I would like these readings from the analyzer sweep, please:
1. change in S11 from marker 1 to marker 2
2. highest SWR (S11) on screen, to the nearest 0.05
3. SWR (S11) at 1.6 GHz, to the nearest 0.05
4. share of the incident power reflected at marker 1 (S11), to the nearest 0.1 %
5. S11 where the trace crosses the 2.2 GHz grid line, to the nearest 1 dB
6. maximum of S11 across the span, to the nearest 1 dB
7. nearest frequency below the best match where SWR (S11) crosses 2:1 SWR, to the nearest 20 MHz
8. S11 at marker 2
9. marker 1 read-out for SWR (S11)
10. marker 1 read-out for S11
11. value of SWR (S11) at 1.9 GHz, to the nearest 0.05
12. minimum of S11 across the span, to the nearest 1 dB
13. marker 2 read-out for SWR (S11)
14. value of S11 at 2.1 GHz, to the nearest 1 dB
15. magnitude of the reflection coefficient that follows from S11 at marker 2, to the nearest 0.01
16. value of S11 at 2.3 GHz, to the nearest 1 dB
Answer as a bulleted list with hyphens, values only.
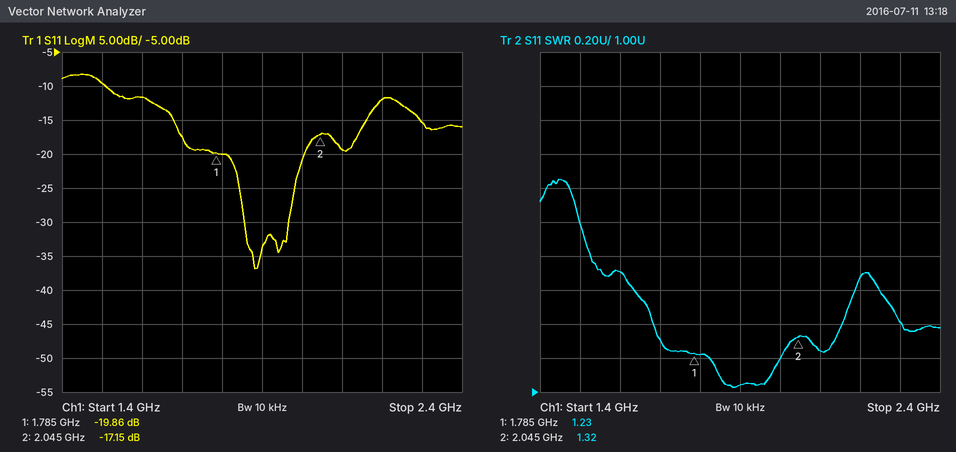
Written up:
- 2.71 dB
- 2.25
- 1.70
- 1.0 %
- -12 dB
- -8 dB
- 1.50 GHz
- -17.15 dB
- 1.23
- -19.86 dB
- 1.05
- -37 dB
- 1.32
- -19 dB
- 0.14
- -15 dB
